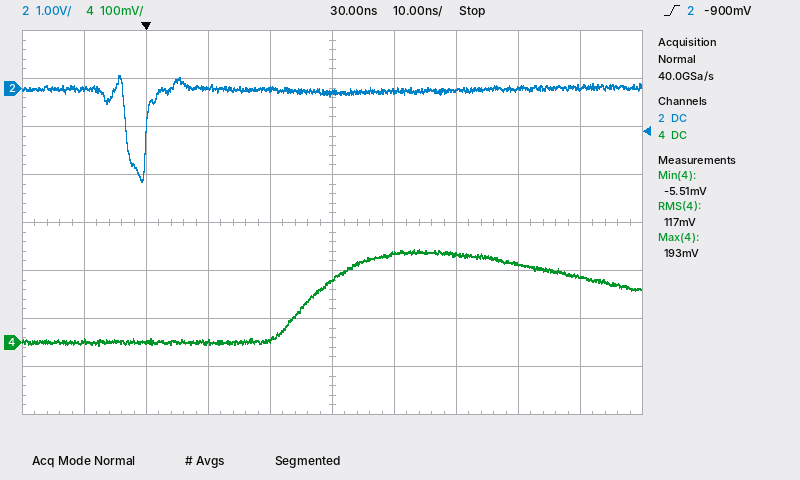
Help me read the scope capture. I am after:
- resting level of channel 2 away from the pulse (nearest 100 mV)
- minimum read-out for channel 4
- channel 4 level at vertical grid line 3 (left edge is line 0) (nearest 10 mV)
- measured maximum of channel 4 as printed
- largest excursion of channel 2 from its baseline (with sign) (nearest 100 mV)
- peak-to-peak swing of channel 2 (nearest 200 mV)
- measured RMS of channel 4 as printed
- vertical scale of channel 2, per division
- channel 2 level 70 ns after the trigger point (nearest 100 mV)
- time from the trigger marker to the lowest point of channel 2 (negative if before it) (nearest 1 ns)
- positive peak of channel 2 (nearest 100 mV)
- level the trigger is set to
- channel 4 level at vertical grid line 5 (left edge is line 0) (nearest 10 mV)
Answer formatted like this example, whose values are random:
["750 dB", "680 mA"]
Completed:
["0.0 V", "-5.51 mV", "0 mV", "193 mV", "-1.9 V", "2.2 V", "117 mV", "1 V", "0.0 V", "-1 ns", "300 mV", "-900 mV", "130 mV"]
